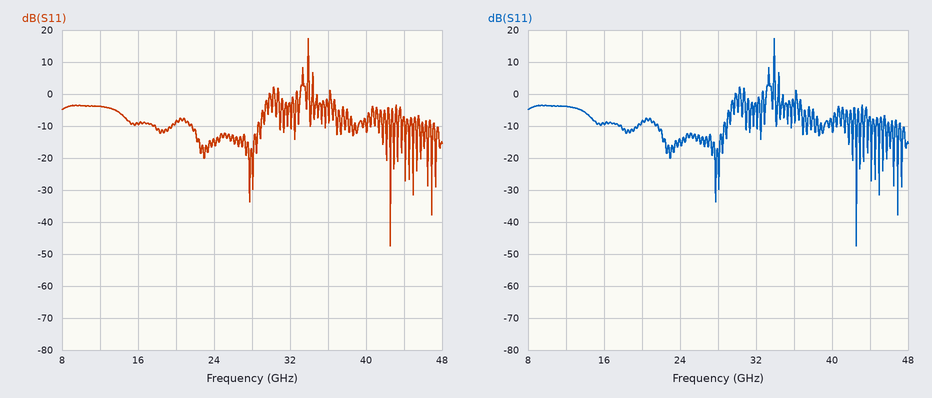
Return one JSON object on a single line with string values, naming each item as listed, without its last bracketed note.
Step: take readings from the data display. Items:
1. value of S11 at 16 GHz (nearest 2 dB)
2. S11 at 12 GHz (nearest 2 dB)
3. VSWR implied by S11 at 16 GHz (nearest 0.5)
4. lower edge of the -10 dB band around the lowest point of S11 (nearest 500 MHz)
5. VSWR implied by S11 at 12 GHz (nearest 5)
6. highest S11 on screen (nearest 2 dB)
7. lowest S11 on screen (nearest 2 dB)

{"value of S11 at 16 GHz": "-10 dB", "S11 at 12 GHz": "-4 dB", "VSWR implied by S11 at 16 GHz": "2.0", "lower edge of the -10 dB band around the lowest point of S11": "42.5 GHz", "VSWR implied by S11 at 12 GHz": "5", "highest S11 on screen": "18 dB", "lowest S11 on screen": "-48 dB"}
